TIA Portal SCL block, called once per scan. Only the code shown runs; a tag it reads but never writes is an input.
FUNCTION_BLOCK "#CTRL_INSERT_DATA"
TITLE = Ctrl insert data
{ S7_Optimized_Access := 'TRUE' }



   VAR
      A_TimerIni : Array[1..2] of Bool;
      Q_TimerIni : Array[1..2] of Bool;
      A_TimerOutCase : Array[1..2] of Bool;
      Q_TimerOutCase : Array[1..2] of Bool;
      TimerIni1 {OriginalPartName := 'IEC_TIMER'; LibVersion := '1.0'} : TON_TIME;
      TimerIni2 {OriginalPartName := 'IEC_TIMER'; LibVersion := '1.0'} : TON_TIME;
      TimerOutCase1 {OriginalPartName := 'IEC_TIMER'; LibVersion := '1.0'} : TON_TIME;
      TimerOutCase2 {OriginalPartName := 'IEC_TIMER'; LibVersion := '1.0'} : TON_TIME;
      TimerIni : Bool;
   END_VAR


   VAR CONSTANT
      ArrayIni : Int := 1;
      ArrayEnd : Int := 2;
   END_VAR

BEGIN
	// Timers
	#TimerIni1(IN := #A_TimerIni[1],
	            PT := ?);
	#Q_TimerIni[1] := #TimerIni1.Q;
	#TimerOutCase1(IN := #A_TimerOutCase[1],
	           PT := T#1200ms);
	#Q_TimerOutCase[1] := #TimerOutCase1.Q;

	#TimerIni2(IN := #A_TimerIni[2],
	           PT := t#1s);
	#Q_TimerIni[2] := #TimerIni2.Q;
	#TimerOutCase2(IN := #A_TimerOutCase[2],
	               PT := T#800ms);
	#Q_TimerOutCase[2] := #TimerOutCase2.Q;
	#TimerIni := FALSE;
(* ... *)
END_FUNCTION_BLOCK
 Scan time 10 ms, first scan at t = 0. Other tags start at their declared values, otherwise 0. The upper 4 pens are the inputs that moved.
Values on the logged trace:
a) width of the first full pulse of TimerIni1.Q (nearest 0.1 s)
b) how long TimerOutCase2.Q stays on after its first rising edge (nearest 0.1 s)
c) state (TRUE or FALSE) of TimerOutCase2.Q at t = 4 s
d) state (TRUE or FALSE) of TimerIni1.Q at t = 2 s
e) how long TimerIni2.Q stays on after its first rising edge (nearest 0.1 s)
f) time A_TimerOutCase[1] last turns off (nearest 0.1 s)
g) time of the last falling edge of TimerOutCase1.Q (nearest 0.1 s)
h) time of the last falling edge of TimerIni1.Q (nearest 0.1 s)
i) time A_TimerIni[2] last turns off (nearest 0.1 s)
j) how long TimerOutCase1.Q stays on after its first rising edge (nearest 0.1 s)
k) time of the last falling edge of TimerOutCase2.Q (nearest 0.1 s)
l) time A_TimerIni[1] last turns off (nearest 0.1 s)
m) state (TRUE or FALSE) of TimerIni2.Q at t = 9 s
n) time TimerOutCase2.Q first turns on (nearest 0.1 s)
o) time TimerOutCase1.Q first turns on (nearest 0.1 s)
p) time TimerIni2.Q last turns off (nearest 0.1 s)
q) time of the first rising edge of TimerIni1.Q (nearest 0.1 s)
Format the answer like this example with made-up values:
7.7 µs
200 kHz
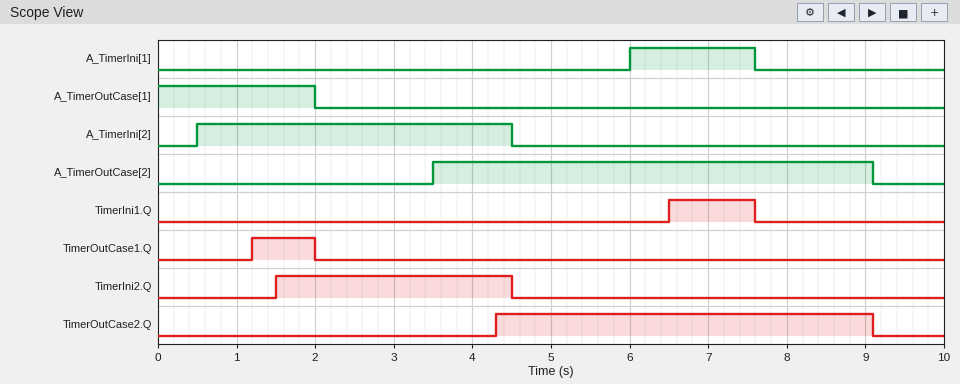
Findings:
1.1 s
4.8 s
FALSE
FALSE
3.0 s
2.0 s
2.0 s
7.6 s
4.5 s
0.8 s
9.1 s
7.6 s
FALSE
4.3 s
1.2 s
4.5 s
6.5 s
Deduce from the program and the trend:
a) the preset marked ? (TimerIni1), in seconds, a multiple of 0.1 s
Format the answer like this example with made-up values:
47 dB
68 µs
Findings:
0.5 s
